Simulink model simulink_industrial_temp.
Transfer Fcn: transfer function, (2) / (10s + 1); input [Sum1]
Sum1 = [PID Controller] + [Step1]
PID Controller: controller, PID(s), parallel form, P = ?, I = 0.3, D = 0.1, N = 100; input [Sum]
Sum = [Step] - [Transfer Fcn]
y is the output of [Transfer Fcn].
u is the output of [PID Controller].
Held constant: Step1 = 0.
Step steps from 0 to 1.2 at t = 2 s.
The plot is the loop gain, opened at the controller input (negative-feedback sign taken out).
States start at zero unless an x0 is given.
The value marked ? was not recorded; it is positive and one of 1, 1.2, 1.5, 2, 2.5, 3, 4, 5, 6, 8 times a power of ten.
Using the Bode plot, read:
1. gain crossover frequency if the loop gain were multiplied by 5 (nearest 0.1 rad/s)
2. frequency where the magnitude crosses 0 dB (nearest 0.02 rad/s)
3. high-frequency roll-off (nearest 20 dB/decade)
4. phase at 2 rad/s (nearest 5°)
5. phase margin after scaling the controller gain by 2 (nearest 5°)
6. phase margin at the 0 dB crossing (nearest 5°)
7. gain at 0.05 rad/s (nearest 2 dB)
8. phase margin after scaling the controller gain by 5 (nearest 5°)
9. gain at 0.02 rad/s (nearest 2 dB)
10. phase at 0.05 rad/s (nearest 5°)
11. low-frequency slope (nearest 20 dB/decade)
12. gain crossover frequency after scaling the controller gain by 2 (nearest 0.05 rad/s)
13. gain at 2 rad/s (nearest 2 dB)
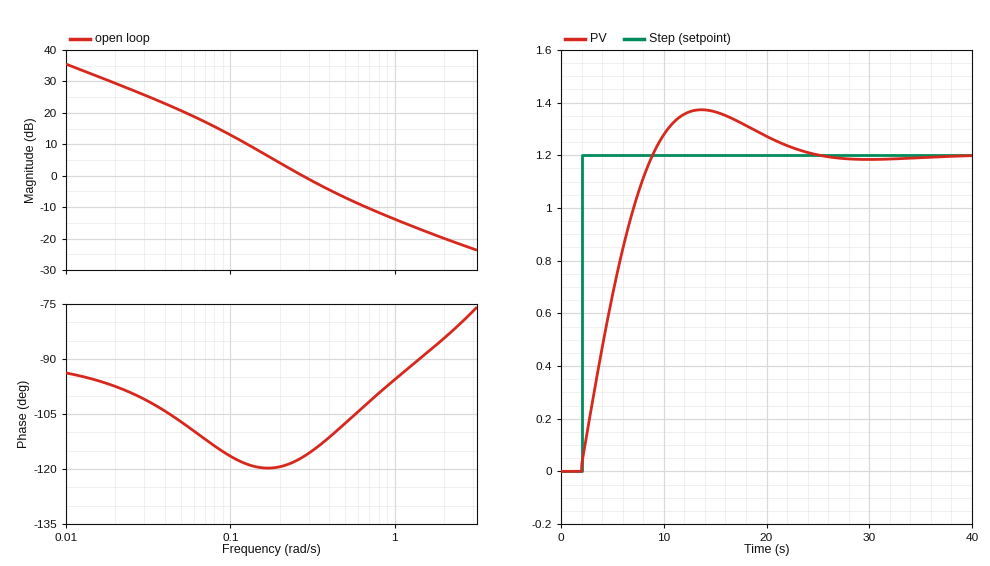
1.0 rad/s
0.28 rad/s
-20 dB/decade
-85°
70°
65°
20 dB
85°
30 dB
-105°
-20 dB/decade
0.45 rad/s
-20 dB
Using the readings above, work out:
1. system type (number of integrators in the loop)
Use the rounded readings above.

1
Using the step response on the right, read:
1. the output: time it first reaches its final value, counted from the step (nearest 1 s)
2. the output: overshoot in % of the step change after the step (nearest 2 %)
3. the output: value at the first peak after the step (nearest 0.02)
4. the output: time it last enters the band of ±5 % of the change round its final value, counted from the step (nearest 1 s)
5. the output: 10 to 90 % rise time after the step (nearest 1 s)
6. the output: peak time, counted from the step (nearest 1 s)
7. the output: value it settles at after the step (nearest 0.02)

7 s
14 %
1.38
19 s
5 s
12 s
1.20
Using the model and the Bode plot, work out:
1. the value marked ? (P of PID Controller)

1
